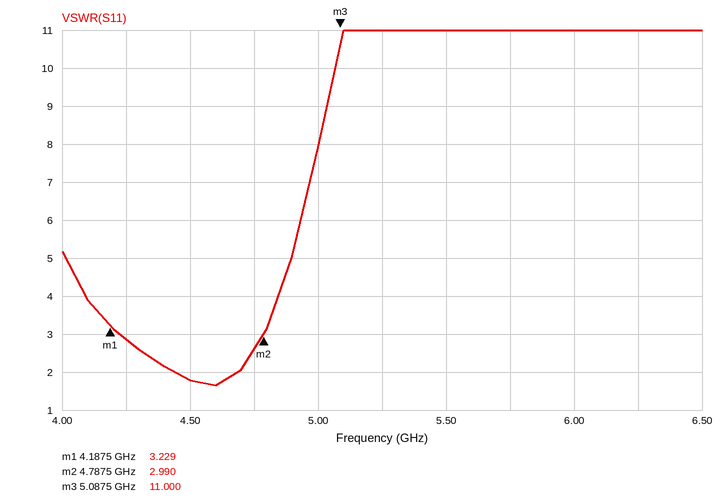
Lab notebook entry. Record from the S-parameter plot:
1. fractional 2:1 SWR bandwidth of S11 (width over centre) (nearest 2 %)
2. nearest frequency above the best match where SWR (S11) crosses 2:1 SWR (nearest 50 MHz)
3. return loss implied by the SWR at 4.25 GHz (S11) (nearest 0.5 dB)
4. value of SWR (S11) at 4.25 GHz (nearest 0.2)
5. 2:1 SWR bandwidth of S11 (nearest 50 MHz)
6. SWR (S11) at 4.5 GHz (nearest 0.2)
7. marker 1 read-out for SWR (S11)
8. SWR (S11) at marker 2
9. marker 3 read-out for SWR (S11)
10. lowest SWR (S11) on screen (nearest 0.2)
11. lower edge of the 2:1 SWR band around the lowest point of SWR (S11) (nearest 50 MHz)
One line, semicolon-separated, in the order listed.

6 %; 4.70 GHz; 6.5 dB; 2.8; 250 MHz; 1.8; 3.229; 2.990; 11.000; 1.6; 4.45 GHz
